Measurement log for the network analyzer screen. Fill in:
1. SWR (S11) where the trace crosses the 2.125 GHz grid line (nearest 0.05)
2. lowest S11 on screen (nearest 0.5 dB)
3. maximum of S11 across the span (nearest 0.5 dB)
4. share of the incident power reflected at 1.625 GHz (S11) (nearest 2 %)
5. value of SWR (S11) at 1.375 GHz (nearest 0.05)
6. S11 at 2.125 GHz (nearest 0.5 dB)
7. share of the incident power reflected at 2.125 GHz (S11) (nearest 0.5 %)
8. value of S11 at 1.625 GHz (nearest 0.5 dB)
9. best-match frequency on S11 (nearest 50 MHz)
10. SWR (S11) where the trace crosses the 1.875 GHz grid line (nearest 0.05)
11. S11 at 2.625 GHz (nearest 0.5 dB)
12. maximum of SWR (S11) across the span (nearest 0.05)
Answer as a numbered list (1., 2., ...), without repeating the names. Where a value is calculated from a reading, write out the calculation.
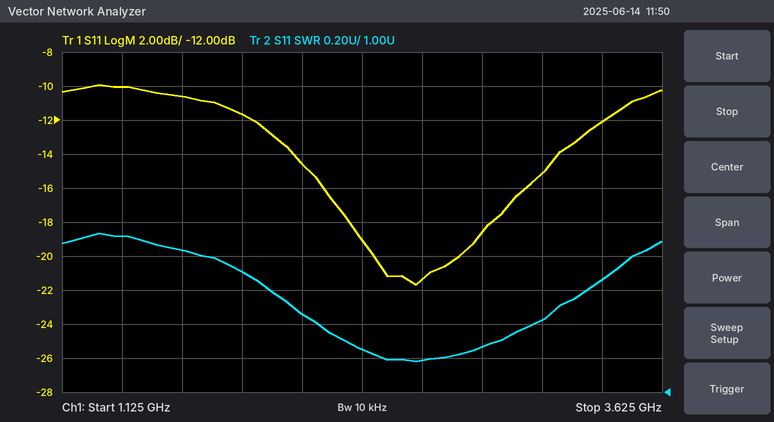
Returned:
1. 1.45
2. -21.5 dB
3. -10.0 dB
4. 10^(-10.5/10) ≈ 8.91 %, so 8 % to the nearest 2 %
5. 1.90
6. -14.5 dB
7. 10^(-14.5/10) ≈ 3.5 %
8. -10.5 dB
9. 2.60 GHz
10. 1.70
11. -21.5 dB
12. 1.95
